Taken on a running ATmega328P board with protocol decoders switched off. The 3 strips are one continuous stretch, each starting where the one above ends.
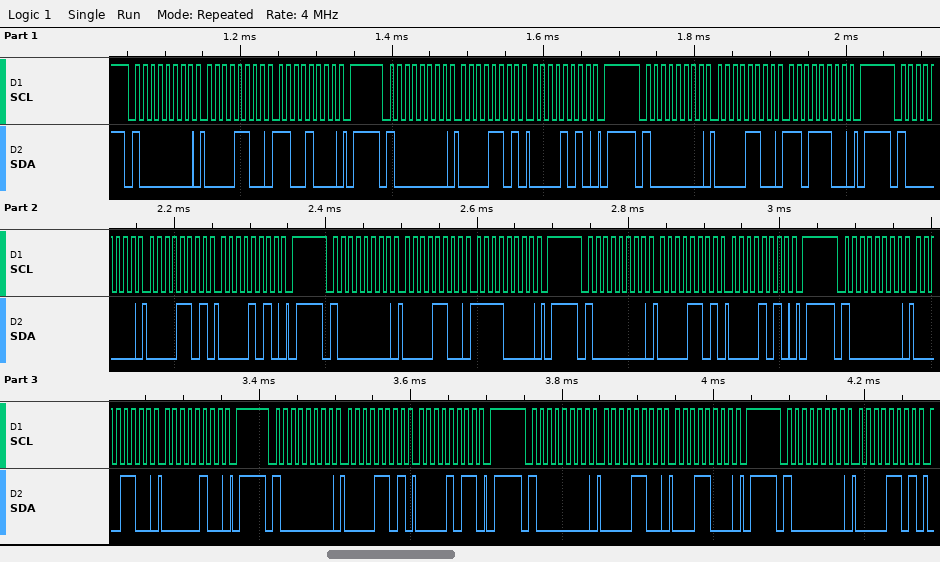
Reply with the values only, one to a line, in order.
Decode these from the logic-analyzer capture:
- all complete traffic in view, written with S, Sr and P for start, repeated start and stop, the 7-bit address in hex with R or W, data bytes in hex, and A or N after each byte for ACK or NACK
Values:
S 40W A 0C A C8 A P S 40W A 0D A 0A A P S 40W A 0C A DC A P S 40W A 0D A 0A A P S 40W A 0C A F0 A P S 40W A 0D A 0A A P S 40W A 0C A 04 A P S 40W A 0D A 0B A P S 40W A 0C A 18 A P S 40W A 0D A
